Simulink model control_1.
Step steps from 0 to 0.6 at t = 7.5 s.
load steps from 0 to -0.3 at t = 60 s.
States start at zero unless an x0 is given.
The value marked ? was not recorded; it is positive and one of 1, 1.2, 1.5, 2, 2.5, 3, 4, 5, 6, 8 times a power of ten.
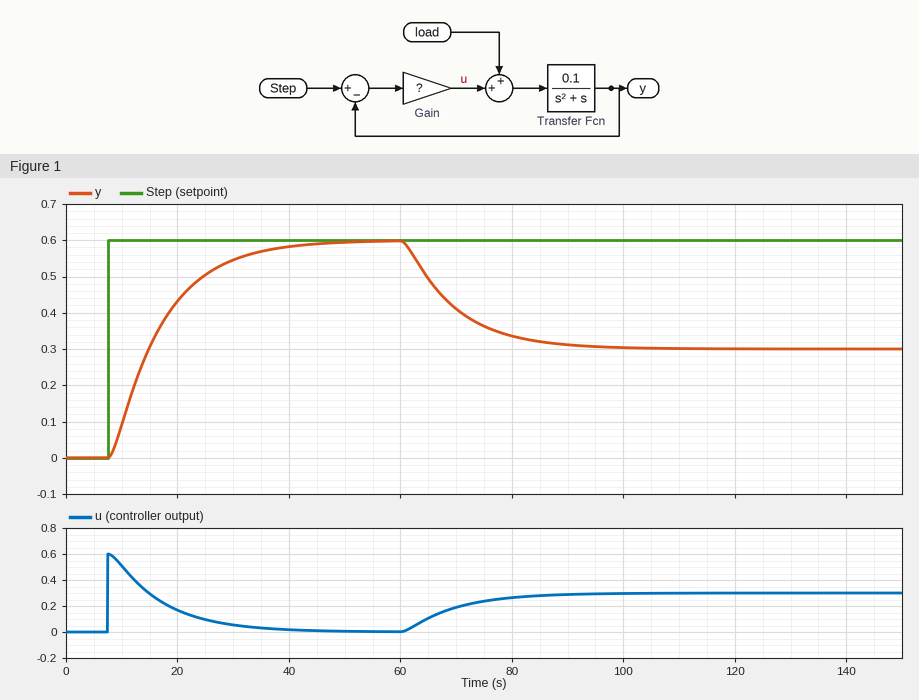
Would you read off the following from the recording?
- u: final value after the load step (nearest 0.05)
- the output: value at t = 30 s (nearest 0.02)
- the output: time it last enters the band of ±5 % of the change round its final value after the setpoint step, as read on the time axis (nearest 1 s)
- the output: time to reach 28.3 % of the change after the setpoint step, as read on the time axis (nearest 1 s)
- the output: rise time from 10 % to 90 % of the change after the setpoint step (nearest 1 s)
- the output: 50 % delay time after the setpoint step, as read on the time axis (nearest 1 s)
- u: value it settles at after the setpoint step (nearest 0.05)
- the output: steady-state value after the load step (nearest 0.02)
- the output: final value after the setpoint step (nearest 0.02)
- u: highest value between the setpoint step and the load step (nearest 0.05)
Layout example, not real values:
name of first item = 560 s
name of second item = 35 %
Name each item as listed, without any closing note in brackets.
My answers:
u: final value after the load step = 0.30
the output: value at t = 30 s = 0.54
the output: time it last enters the band of ±5 % of the change round its final value after the setpoint step, as read on the time axis = 35 s
the output: time to reach 28.3 % of the change after the setpoint step, as read on the time axis = 12 s
the output: rise time from 10 % to 90 % of the change after the setpoint step = 20 s
the output: 50 % delay time after the setpoint step, as read on the time axis = 15 s
u: value it settles at after the setpoint step = 0.00
the output: steady-state value after the load step = 0.30
the output: final value after the setpoint step = 0.60
u: highest value between the setpoint step and the load step = 0.60
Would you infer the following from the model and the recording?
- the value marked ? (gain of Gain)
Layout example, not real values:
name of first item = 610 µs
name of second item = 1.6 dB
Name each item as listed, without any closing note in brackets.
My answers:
the value marked ? = 1
